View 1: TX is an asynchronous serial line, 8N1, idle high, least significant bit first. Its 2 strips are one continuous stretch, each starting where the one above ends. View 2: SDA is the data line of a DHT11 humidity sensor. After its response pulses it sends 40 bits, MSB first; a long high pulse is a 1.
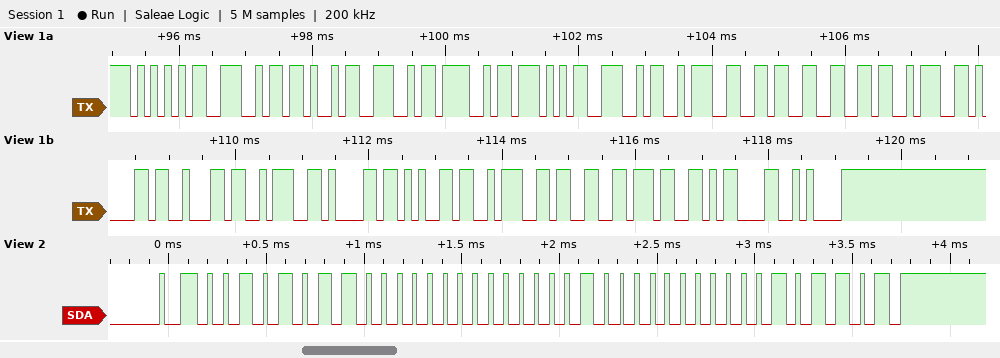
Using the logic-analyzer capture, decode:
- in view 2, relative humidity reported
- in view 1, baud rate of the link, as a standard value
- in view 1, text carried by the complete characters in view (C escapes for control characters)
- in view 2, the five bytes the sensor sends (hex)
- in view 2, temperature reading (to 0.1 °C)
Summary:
43 %
9600 baud
"UNKNOWN:6f:ab:ae:37\r\n"
2B 00 02 00 2D
2.0 °C
